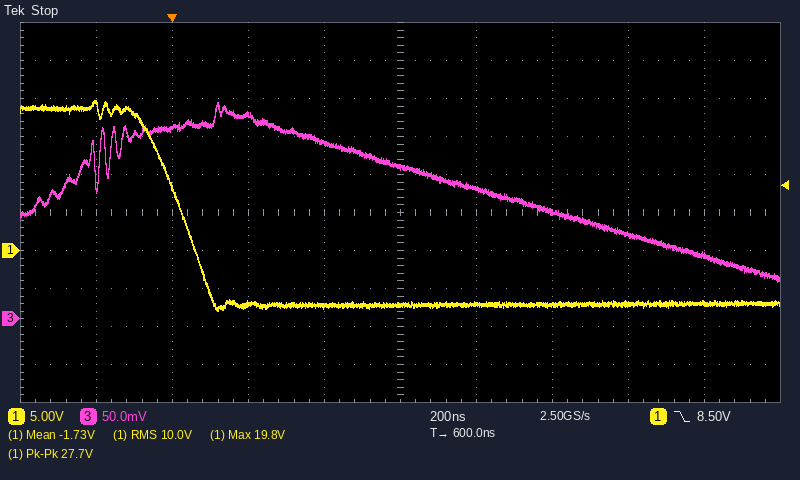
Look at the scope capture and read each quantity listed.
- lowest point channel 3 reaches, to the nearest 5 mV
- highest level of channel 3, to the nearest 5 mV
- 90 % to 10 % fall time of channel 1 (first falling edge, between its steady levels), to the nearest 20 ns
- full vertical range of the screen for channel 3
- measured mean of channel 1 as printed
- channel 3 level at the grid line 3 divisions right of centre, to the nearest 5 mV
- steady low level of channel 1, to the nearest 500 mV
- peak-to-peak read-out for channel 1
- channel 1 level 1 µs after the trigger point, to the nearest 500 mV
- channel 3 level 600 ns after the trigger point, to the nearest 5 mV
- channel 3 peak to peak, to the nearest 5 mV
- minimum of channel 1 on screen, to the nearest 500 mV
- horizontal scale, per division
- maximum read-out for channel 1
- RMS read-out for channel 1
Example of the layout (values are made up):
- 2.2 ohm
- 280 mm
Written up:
- 50 mV
- 285 mV
- 160 ns
- 500 mV
- -1.73 V
- 110 mV
- -7.0 V
- 27.7 V
- -7.0 V
- 200 mV
- 235 mV
- -8.0 V
- 200 ns
- 19.8 V
- 10.0 V
